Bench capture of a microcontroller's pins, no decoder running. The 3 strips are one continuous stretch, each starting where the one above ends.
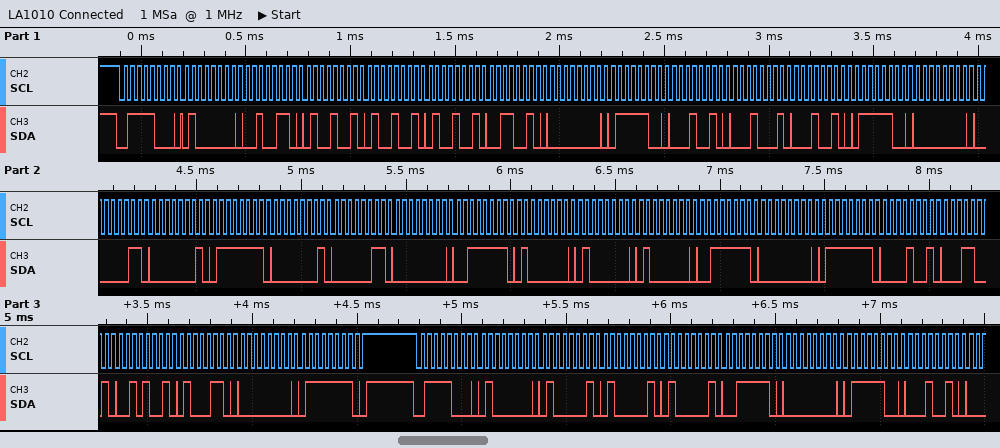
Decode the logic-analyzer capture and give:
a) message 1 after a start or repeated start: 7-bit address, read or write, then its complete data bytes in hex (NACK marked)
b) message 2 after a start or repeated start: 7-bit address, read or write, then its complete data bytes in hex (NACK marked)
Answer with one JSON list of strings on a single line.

["0x3C write: 40 26 49 49 49 32 00 7C 12 11 12 7C 00 03 01 7F 01 03 00 3F 40 40 40 3F 00 7F 09 19 29 46 00 7F", "0x3C write: 40 41 41 41 3E 00 7C 12"]
